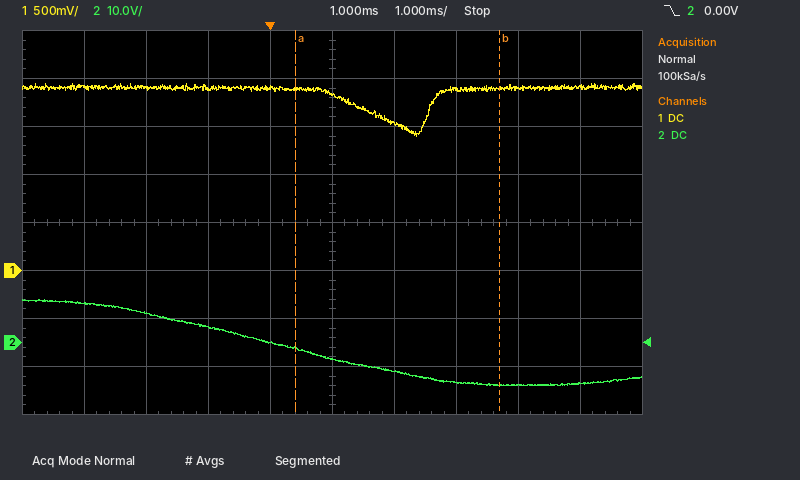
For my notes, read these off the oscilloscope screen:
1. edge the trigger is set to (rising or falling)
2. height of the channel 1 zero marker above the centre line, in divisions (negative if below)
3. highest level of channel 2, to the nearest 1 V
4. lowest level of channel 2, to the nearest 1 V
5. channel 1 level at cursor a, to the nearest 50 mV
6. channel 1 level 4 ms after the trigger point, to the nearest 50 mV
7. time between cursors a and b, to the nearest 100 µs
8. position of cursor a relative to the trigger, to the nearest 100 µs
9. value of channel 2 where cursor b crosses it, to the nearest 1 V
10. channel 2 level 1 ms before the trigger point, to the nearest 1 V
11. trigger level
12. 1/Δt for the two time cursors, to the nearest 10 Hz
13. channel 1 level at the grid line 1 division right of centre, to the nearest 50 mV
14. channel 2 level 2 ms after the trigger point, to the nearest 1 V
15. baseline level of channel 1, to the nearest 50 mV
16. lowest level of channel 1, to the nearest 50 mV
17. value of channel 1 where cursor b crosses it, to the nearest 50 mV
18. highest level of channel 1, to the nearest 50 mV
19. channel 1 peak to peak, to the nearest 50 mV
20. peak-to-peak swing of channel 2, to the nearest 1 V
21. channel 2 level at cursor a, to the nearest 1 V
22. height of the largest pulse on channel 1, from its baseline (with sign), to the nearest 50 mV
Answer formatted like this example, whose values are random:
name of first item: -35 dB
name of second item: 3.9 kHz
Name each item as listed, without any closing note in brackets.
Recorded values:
edge the trigger is set to: falling
height of the channel 1 zero marker above the centre line, in divisions: -1.0 div
highest level of channel 2, to the nearest 1 V: 9 V
lowest level of channel 2, to the nearest 1 V: -9 V
channel 1 level at cursor a, to the nearest 50 mV: 1.90 V
channel 1 level 4 ms after the trigger point, to the nearest 50 mV: 1.90 V
time between cursors a and b, to the nearest 100 µs: 3.3 ms
position of cursor a relative to the trigger, to the nearest 100 µs: +400 µs
value of channel 2 where cursor b crosses it, to the nearest 1 V: -9 V
channel 2 level 1 ms before the trigger point, to the nearest 1 V: 3 V
trigger level: 0.00 V
1/Δt for the two time cursors, to the nearest 10 Hz: 300 Hz
channel 1 level at the grid line 1 division right of centre, to the nearest 50 mV: 1.55 V
channel 2 level 2 ms after the trigger point, to the nearest 1 V: -6 V
baseline level of channel 1, to the nearest 50 mV: 1.90 V
lowest level of channel 1, to the nearest 50 mV: 1.40 V
value of channel 1 where cursor b crosses it, to the nearest 50 mV: 1.90 V
highest level of channel 1, to the nearest 50 mV: 1.95 V
channel 1 peak to peak, to the nearest 50 mV: 550 mV
peak-to-peak swing of channel 2, to the nearest 1 V: 18 V
channel 2 level at cursor a, to the nearest 1 V: -1 V
height of the largest pulse on channel 1, from its baseline (with sign), to the nearest 50 mV: -500 mV
